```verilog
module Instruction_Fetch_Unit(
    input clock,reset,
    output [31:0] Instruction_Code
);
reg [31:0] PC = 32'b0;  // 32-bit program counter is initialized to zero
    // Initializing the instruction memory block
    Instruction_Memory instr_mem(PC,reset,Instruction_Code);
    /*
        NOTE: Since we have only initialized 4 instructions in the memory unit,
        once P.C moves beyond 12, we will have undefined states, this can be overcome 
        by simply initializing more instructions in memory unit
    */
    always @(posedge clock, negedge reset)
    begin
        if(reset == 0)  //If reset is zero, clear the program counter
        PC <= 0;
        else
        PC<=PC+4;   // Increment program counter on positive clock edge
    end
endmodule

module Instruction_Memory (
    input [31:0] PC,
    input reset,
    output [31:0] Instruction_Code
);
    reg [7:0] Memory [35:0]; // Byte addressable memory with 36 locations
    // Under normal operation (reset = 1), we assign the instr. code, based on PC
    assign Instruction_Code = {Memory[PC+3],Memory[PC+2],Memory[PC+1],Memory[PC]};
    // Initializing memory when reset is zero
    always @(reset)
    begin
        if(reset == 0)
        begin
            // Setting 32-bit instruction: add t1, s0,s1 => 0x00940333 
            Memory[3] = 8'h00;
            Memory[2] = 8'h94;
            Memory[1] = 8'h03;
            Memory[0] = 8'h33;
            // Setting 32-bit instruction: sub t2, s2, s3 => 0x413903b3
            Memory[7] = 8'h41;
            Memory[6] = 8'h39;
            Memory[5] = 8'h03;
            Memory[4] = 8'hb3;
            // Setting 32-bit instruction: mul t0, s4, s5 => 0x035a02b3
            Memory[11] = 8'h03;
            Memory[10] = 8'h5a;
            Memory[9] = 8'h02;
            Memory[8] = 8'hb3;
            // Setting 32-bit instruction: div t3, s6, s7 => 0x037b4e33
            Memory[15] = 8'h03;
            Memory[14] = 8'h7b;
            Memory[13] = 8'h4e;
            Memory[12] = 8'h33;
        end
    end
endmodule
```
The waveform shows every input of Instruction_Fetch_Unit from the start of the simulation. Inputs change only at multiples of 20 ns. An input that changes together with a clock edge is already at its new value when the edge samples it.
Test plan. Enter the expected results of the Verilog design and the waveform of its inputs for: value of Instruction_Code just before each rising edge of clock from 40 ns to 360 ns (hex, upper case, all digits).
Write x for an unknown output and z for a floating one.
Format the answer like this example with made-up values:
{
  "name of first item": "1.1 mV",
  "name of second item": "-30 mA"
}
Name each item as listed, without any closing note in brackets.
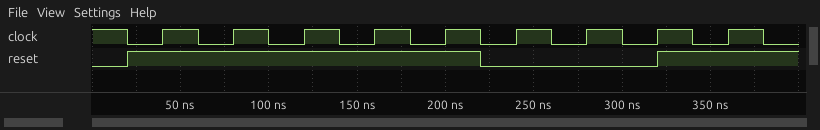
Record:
{
  "value of Instruction_Code just before each rising edge of clock from 40 ns to 360 ns": "00940333, 413903B3, 035A02B3, 037B4E33, x, 00940333, 00940333, 00940333, 413903B3"
}
